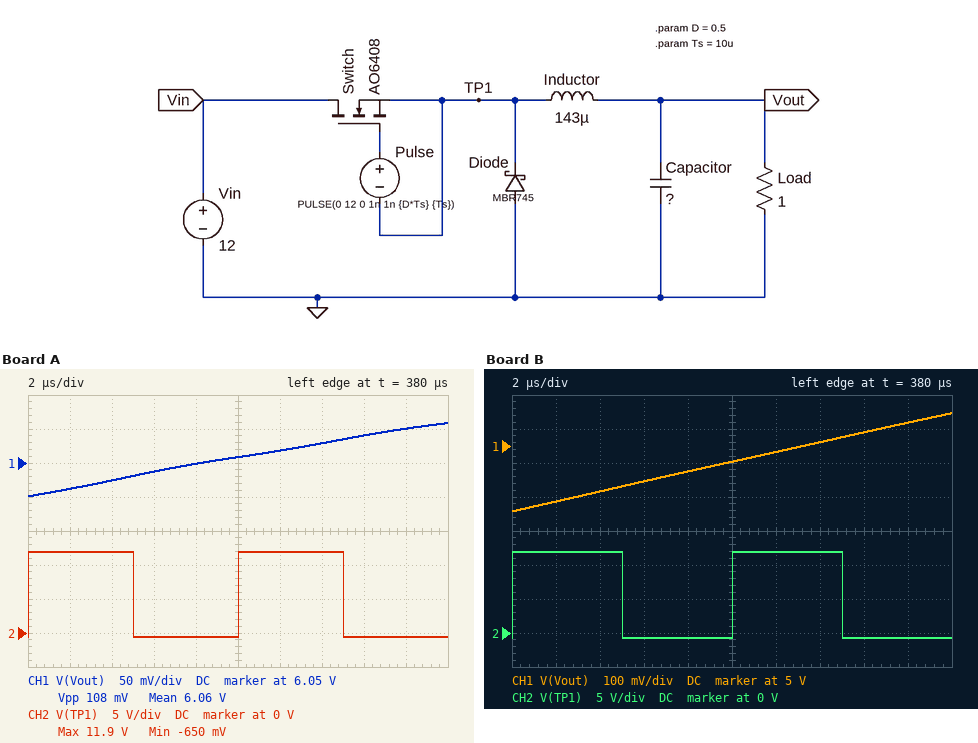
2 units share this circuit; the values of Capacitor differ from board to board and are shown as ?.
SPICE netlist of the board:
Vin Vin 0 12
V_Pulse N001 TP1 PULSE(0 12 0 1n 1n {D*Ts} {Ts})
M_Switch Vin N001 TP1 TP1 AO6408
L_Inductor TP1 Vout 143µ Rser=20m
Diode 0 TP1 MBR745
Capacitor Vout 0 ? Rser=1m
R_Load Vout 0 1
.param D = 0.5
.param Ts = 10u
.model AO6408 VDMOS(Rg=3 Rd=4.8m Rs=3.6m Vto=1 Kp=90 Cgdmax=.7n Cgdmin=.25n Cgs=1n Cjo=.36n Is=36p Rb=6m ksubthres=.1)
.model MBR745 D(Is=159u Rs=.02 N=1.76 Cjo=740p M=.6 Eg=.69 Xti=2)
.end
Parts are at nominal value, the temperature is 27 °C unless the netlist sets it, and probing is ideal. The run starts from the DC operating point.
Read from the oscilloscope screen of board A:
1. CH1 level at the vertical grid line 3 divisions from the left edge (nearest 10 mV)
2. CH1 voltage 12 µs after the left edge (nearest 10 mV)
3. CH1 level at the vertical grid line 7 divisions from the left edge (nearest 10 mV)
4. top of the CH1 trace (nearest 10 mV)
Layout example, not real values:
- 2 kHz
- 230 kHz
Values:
- 6.04 V
- 6.07 V
- 6.08 V
- 6.11 V
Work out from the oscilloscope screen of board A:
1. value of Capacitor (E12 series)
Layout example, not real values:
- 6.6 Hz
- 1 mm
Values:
- 120 µF
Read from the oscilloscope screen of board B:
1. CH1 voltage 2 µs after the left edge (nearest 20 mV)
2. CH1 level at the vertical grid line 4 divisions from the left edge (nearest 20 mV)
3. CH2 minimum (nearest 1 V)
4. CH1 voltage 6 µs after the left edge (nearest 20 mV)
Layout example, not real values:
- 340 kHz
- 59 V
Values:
- 4.84 V
- 4.92 V
- -1 V
- 4.90 V
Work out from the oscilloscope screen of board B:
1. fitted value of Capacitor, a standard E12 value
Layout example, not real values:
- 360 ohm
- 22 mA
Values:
- 330 µF
